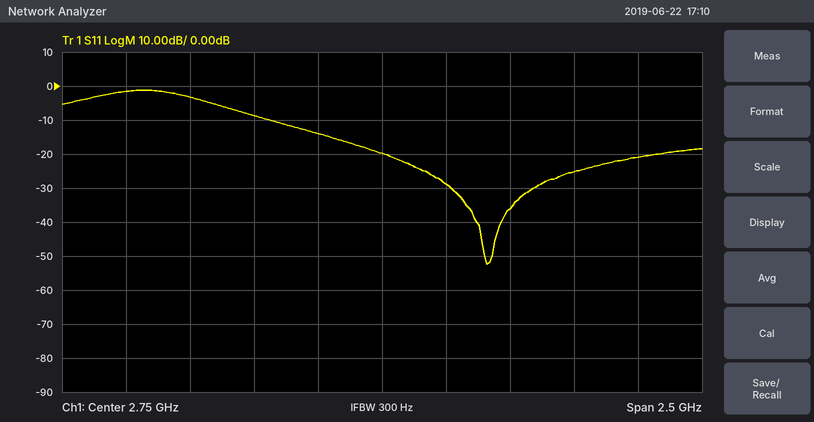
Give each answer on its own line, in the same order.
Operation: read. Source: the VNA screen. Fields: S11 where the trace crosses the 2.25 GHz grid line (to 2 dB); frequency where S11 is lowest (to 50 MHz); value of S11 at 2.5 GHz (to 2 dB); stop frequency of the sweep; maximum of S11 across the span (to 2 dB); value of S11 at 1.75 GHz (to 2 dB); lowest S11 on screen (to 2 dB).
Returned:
-8 dB
3.15 GHz
-14 dB
4 GHz
-2 dB
-2 dB
-52 dB
